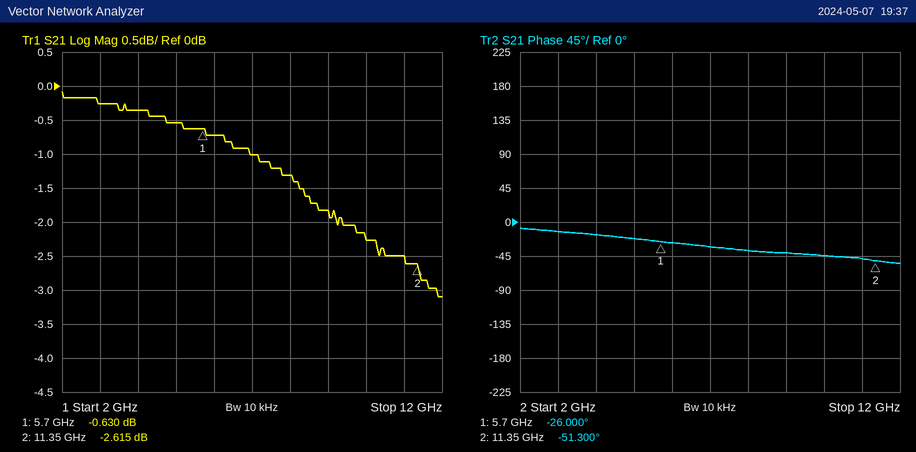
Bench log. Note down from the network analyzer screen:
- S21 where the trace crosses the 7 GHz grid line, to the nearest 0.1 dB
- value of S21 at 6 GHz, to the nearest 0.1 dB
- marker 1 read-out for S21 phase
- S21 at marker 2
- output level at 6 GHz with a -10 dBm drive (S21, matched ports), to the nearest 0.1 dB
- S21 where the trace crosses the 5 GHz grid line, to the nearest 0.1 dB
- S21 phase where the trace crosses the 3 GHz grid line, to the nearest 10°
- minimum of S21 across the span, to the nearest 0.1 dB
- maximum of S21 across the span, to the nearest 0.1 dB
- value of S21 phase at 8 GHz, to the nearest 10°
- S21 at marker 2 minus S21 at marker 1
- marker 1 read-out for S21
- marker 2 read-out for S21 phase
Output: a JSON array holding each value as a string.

["-1.0 dB", "-0.7 dB", "-26.000°", "-2.615 dB", "-10.7 dBm", "-0.5 dB", "-10°", "-3.1 dB", "-0.1 dB", "-40°", "-1.985 dB", "-0.630 dB", "-51.300°"]
